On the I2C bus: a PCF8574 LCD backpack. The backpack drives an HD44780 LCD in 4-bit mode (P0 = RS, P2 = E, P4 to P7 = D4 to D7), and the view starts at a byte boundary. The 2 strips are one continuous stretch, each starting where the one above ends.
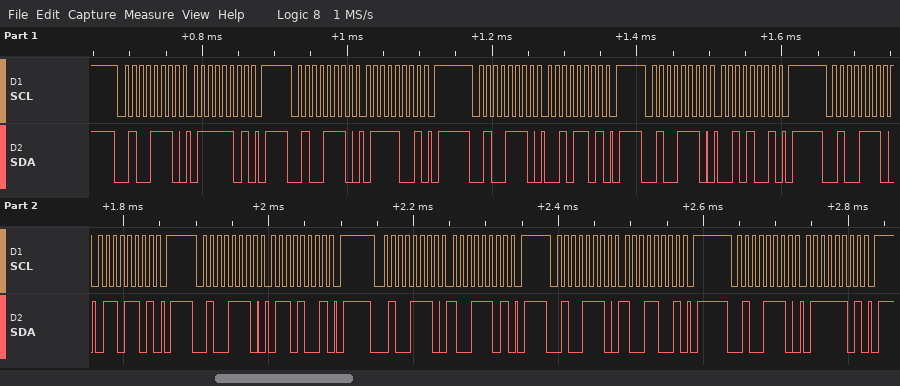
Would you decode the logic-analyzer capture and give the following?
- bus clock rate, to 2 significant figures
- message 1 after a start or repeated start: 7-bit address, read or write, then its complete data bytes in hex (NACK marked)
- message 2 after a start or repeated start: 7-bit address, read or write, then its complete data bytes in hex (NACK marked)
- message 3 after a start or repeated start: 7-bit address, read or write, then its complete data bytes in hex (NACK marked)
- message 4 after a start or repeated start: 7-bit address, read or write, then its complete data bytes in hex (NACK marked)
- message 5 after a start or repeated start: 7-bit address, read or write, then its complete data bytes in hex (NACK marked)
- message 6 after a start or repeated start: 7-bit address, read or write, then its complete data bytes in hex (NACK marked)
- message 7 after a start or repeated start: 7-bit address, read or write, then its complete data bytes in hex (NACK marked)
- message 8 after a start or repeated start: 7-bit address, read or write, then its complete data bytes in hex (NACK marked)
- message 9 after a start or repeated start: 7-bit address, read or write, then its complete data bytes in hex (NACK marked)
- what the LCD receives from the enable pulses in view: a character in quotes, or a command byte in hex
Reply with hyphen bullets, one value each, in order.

- 100 kHz
- 0x27 write: 7D
- 0x27 write: 79
- 0x27 write: 2D
- 0x27 write: 29
- 0x27 write: 6D
- 0x27 write: 69
- 0x27 write: 9D
- 0x27 write: 99
- 0x27 write: 7D
- 'r' 'i'
